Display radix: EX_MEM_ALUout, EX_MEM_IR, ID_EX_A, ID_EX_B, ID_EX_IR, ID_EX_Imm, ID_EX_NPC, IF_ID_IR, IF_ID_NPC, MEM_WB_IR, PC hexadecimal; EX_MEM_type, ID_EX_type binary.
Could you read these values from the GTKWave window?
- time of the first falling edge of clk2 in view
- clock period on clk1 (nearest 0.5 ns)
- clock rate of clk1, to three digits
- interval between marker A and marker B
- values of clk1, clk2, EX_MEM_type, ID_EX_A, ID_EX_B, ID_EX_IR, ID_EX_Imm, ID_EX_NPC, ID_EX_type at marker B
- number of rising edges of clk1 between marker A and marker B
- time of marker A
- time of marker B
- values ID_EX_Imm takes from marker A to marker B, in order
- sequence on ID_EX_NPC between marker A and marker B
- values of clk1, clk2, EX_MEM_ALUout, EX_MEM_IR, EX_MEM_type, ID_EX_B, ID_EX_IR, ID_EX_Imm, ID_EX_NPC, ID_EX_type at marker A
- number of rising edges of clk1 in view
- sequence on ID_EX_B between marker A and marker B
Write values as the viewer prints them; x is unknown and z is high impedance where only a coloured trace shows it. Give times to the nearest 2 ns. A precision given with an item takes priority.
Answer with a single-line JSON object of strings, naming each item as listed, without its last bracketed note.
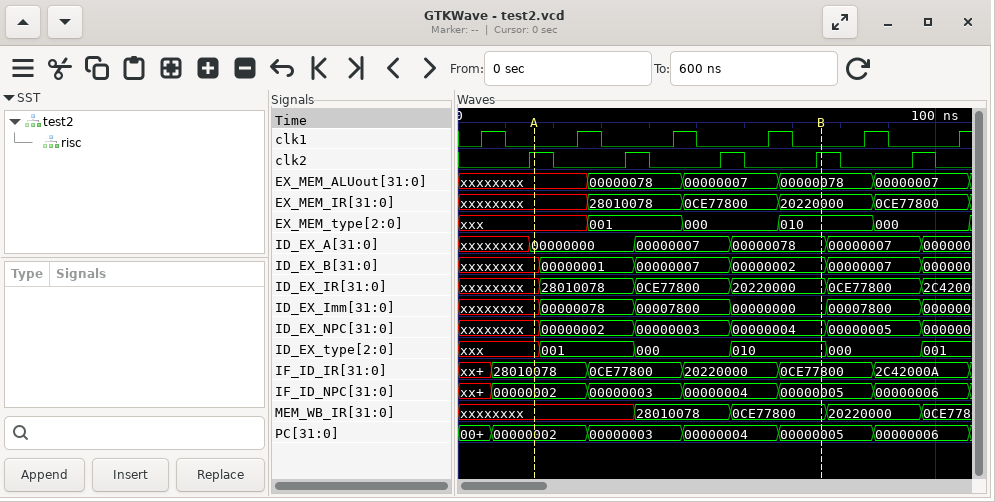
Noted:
{"time of the first falling edge of clk2 in view": "20 ns", "clock period on clk1": "20 ns", "clock rate of clk1, to three digits": "50.0 MHz", "interval between marker A and marker B": "60 ns", "values of clk1, clk2, EX_MEM_type, ID_EX_A, ID_EX_B, ID_EX_IR, ID_EX_Imm, ID_EX_NPC, ID_EX_type at marker B": "clk1=0, clk2=1, EX_MEM_type=010, ID_EX_A=00000078, ID_EX_B=00000002, ID_EX_IR=20220000, ID_EX_Imm=00000000, ID_EX_NPC=00000004, ID_EX_type=010", "number of rising edges of clk1 between marker A and marker B": "3", "time of marker A": "16 ns", "time of marker B": "76 ns", "values ID_EX_Imm takes from marker A to marker B, in order": "xxxxxxxx, 00000078, 00007800, 00000000", "sequence on ID_EX_NPC between marker A and marker B": "xxxxxxxx, 00000002, 00000003, 00000004", "values of clk1, clk2, EX_MEM_ALUout, EX_MEM_IR, EX_MEM_type, ID_EX_B, ID_EX_IR, ID_EX_Imm, ID_EX_NPC, ID_EX_type at marker A": "clk1=0, clk2=1, EX_MEM_ALUout=xxxxxxxx, EX_MEM_IR=xxxxxxxx, EX_MEM_type=xxx, ID_EX_B=xxxxxxxx, ID_EX_IR=xxxxxxxx, ID_EX_Imm=xxxxxxxx, ID_EX_NPC=xxxxxxxx, ID_EX_type=xxx", "number of rising edges of clk1 in view": "6", "sequence on ID_EX_B between marker A and marker B": "xxxxxxxx, 00000001, 00000007, 00000002"}
